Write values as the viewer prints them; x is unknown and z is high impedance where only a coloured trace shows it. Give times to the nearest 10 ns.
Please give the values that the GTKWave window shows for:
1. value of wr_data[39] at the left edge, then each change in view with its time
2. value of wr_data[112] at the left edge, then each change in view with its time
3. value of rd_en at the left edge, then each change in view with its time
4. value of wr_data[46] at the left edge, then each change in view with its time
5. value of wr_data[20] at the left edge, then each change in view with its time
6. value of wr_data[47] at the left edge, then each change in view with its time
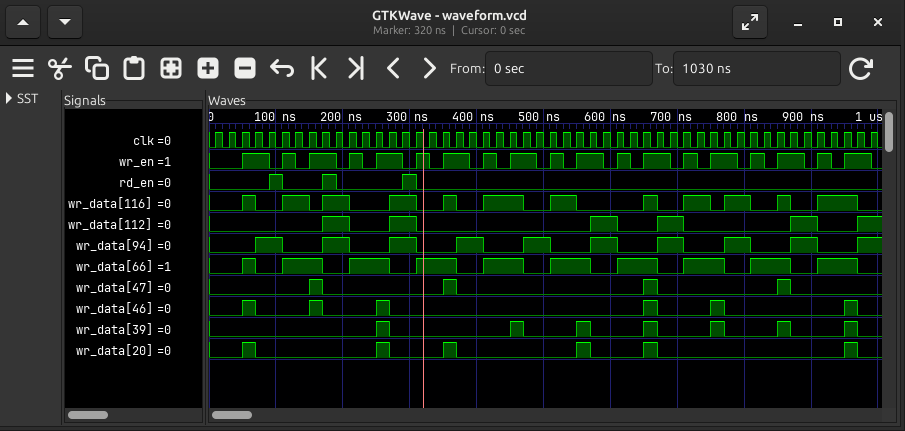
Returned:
0, 1 at 250 ns, 0 at 270 ns, 1 at 450 ns, 0 at 470 ns, 1 at 550 ns, 0 at 570 ns, 1 at 650 ns, 0 at 670 ns, 1 at 750 ns, 0 at 770 ns, 1 at 850 ns, 0 at 870 ns, 1 at 950 ns, 0 at 970 ns
0, 1 at 170 ns, 0 at 210 ns, 1 at 270 ns, 0 at 310 ns, 1 at 570 ns, 0 at 610 ns, 1 at 670 ns, 0 at 710 ns, 1 at 870 ns, 0 at 910 ns, 1 at 970 ns
0, 1 at 90 ns, 0 at 110 ns, 1 at 170 ns, 0 at 190 ns, 1 at 290 ns, 0 at 310 ns
0, 1 at 50 ns, 0 at 70 ns, 1 at 150 ns, 0 at 170 ns, 1 at 250 ns, 0 at 270 ns, 1 at 650 ns, 0 at 670 ns, 1 at 750 ns, 0 at 770 ns, 1 at 950 ns, 0 at 970 ns
0, 1 at 50 ns, 0 at 70 ns, 1 at 250 ns, 0 at 270 ns, 1 at 350 ns, 0 at 370 ns, 1 at 550 ns, 0 at 570 ns, 1 at 650 ns, 0 at 670 ns, 1 at 950 ns, 0 at 970 ns
0, 1 at 150 ns, 0 at 170 ns, 1 at 350 ns, 0 at 370 ns, 1 at 650 ns, 0 at 670 ns, 1 at 850 ns, 0 at 870 ns
